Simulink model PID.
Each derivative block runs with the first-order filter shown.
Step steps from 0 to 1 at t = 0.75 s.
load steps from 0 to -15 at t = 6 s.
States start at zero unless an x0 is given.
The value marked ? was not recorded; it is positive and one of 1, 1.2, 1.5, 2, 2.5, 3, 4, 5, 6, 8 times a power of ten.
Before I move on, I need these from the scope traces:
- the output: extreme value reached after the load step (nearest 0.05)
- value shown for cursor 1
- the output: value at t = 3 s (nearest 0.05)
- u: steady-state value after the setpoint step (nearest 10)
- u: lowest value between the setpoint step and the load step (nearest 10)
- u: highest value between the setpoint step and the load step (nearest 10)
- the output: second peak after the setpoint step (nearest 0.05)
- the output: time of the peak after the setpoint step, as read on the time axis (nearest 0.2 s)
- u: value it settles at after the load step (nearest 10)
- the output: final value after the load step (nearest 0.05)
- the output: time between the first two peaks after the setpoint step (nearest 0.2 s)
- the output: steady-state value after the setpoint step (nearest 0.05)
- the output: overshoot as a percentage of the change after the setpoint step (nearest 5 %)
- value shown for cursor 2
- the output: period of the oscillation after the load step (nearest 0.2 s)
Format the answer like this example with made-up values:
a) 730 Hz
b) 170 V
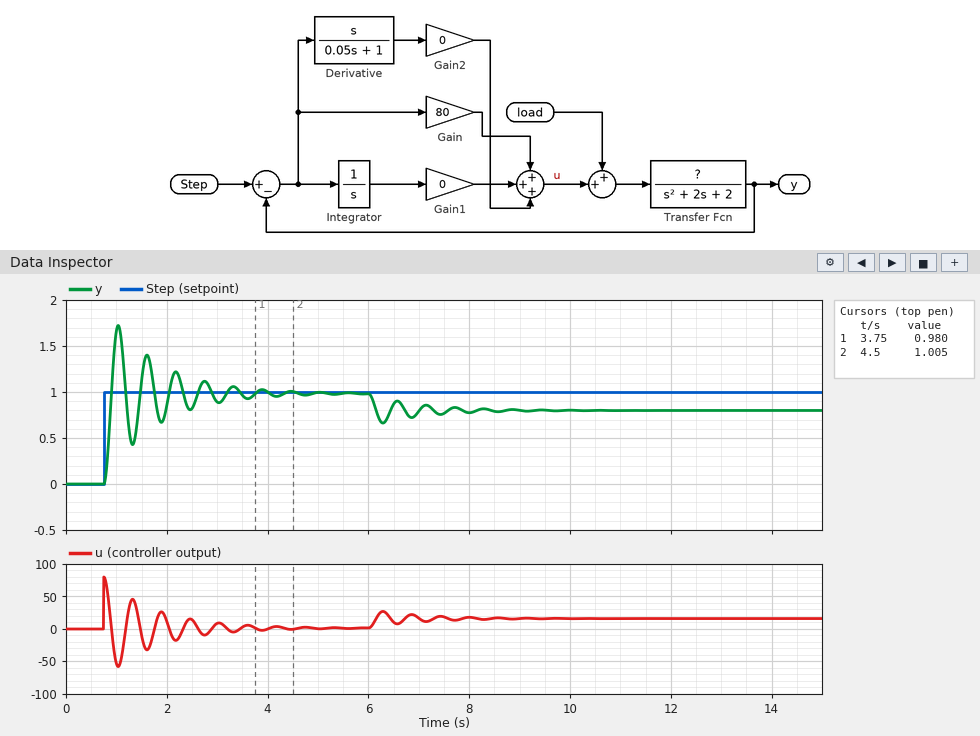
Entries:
a) 0.65
b) 0.980
c) 0.90
d) 0
e) -60
f) 80
g) 1.40
h) 1.0 s
i) 20
j) 0.80
k) 0.6 s
l) 1.00
m) 75 %
n) 1.005
o) 0.6 s
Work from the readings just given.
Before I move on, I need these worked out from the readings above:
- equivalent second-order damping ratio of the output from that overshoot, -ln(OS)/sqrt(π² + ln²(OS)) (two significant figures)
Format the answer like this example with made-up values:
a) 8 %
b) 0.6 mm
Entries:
a) 0.091
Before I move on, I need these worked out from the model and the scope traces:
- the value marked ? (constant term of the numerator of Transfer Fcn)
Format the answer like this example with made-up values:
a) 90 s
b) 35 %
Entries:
a) 1.5
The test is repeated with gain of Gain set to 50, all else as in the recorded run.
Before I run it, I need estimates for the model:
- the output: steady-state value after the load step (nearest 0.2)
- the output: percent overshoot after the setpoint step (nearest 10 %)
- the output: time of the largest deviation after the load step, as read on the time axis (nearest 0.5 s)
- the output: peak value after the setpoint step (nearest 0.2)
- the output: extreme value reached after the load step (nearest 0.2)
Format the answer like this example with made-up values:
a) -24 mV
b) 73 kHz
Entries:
a) 0.6
b) 70 %
c) 6.5 s
d) 1.6
e) 0.4
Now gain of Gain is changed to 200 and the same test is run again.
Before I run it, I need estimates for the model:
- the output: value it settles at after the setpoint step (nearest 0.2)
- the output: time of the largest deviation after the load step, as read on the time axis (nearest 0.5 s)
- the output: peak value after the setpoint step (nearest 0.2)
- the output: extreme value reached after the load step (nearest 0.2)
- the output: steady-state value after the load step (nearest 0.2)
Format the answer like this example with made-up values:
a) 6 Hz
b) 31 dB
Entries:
a) 1.0
b) 6.0 s
c) 1.8
d) 0.8
e) 1.0
